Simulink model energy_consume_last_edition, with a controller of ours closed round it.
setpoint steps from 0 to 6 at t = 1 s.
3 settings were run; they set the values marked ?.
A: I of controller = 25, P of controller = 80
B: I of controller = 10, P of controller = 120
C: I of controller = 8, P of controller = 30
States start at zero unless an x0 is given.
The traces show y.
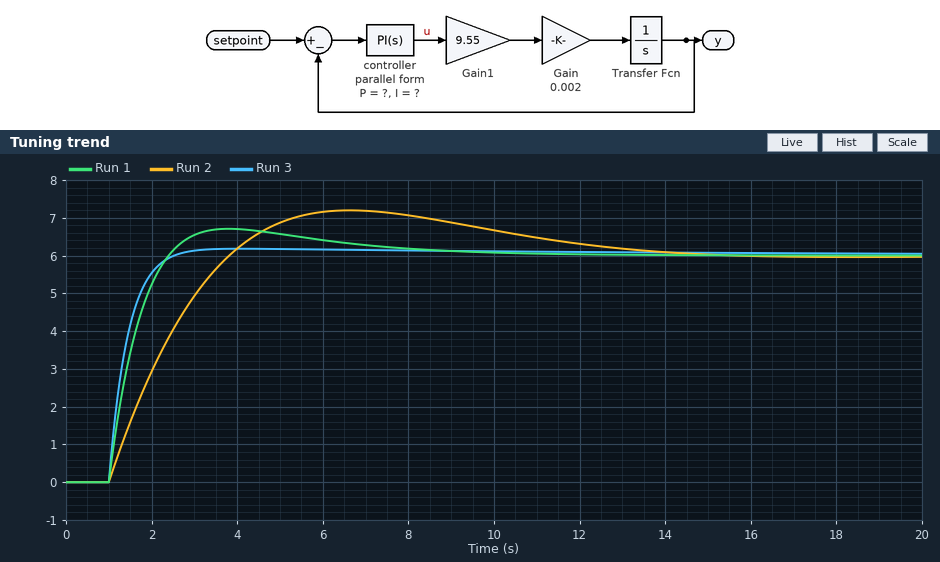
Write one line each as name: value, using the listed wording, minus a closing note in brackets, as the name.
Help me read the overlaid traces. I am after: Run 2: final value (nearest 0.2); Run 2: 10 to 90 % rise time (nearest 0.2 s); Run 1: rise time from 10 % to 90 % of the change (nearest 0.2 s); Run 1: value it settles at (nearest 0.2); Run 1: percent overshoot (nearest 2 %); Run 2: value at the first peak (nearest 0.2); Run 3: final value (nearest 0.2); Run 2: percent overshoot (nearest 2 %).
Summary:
Run 2: final value: 6.0
Run 2: 10 to 90 % rise time: 2.2 s
Run 1: rise time from 10 % to 90 % of the change: 1.0 s
Run 1: value it settles at: 6.0
Run 1: percent overshoot: 12 %
Run 2: value at the first peak: 7.2
Run 3: final value: 6.0
Run 2: percent overshoot: 20 %
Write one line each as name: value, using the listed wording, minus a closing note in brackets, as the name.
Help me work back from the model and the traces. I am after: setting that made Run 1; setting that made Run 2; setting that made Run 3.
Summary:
setting that made Run 1: A
setting that made Run 2: C
setting that made Run 3: B
